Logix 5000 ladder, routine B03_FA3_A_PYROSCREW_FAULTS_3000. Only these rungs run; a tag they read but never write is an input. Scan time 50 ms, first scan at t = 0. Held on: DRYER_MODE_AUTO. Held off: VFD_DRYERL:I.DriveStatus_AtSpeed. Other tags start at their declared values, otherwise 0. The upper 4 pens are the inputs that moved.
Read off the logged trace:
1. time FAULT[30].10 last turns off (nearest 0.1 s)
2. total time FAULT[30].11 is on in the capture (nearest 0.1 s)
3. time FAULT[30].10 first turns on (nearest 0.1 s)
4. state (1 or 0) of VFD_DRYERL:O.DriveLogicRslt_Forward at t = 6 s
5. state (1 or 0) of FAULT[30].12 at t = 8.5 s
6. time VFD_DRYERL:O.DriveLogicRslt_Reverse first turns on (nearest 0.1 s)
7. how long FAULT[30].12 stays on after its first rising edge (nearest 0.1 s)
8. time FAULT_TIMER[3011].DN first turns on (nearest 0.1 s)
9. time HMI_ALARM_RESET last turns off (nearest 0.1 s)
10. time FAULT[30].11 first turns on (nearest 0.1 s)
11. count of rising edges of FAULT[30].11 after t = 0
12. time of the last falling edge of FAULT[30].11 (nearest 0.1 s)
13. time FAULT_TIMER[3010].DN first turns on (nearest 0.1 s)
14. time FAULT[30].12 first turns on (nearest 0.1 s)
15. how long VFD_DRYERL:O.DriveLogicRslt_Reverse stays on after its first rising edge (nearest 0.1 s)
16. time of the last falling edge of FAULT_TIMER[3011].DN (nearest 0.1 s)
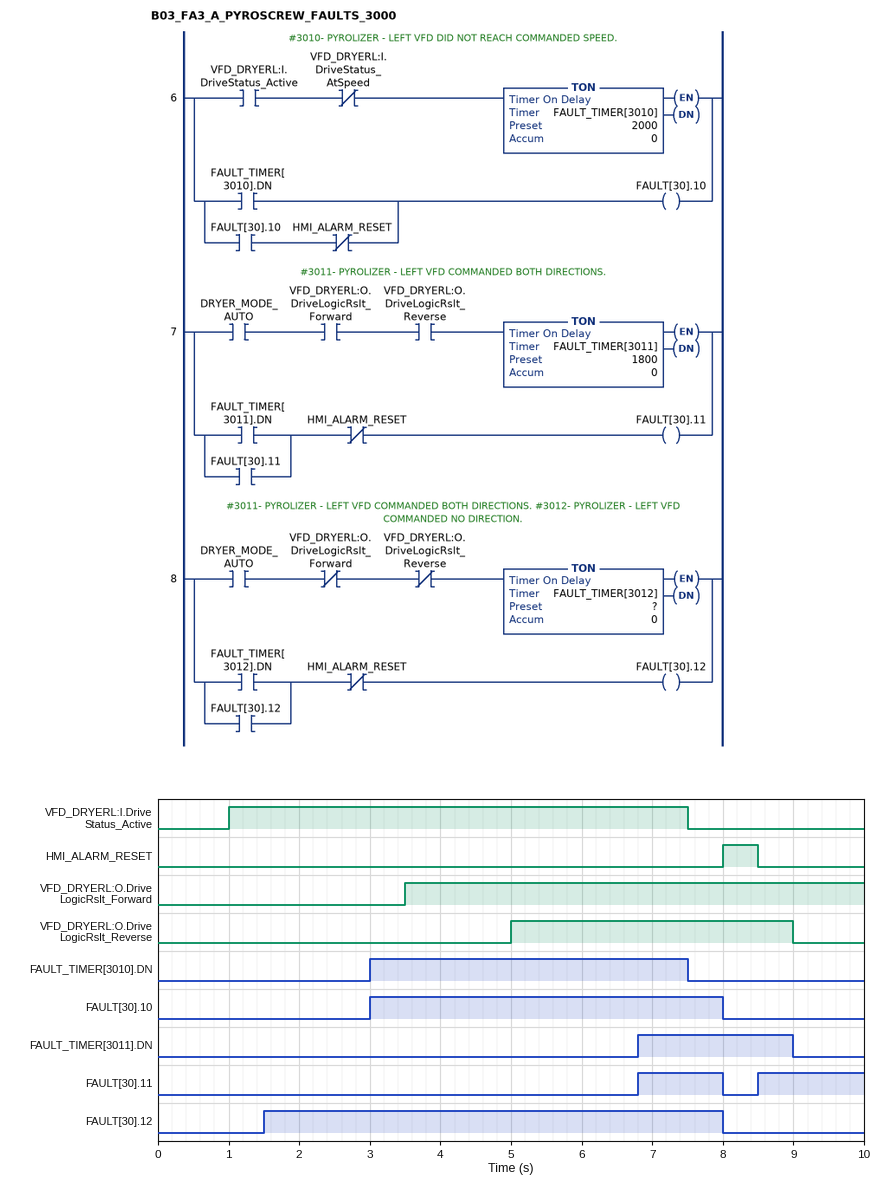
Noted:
8.0 s
2.7 s
3.0 s
1
0
5.0 s
6.5 s
6.8 s
8.5 s
6.8 s
2
8.0 s
3.0 s
1.5 s
4.0 s
9.0 s
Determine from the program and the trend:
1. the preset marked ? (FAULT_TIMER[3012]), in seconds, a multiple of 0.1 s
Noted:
1.5 s
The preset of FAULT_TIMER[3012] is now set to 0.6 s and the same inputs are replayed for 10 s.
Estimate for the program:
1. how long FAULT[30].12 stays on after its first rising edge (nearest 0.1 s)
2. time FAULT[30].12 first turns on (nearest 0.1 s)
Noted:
7.4 s
0.6 s
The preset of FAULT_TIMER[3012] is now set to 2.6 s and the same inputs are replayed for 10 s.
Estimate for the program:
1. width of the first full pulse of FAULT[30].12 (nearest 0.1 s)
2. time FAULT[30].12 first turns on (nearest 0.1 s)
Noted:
5.4 s
2.6 s
